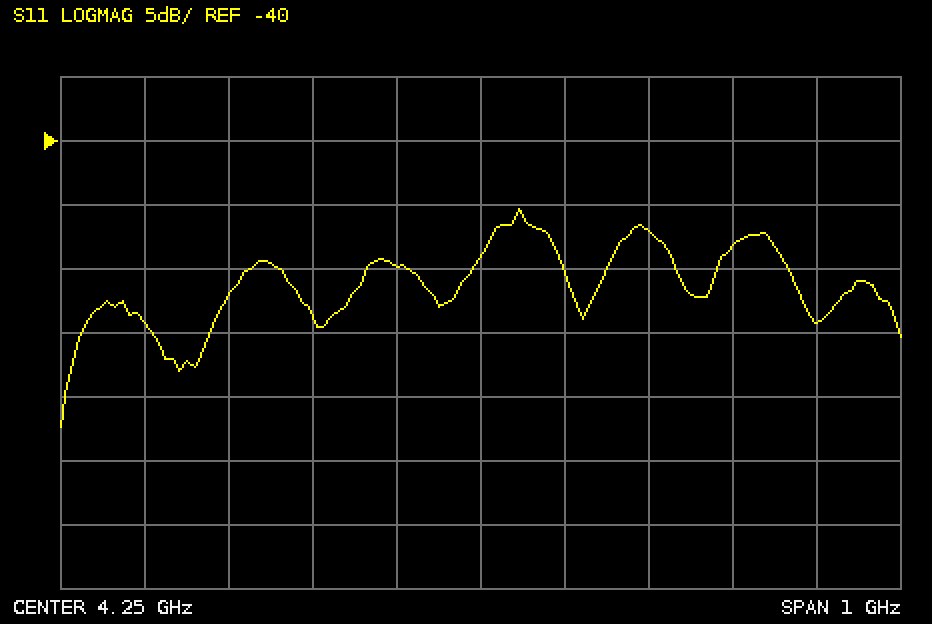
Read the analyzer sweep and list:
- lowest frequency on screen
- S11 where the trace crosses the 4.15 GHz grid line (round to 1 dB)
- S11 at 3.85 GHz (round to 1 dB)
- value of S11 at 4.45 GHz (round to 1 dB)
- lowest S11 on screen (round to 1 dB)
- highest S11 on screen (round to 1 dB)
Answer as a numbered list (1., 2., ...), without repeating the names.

1. 3.75 GHz
2. -50 dB
3. -54 dB
4. -47 dB
5. -62 dB
6. -45 dB
